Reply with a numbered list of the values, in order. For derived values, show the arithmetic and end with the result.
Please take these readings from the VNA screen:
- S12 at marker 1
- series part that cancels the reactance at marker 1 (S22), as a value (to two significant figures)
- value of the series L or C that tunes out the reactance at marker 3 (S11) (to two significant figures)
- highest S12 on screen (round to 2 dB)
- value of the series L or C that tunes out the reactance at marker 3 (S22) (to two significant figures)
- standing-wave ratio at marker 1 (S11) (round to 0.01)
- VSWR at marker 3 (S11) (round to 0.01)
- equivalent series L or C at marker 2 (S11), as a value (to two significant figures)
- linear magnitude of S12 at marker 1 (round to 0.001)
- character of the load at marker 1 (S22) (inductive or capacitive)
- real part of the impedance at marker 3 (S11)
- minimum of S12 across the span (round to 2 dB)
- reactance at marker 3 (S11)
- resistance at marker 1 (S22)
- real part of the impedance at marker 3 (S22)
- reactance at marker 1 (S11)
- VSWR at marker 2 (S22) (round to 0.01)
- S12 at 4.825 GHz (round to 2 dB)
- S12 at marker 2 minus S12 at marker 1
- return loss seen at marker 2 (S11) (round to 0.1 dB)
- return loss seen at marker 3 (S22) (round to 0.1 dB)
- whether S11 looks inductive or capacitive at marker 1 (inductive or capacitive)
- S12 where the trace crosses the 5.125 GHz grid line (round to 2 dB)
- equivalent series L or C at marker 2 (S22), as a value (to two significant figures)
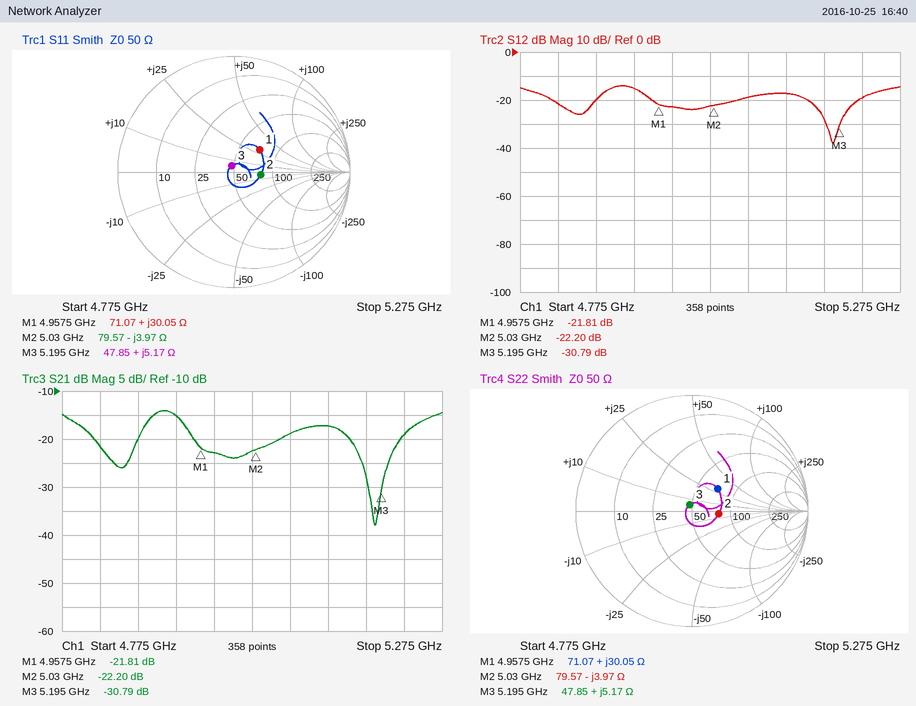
1. -21.81 dB
2. C = 1/(2π × 4.9575 GHz × 30.05 Ω) ≈ 1.1 pF
3. C = 1/(2π × 5.195 GHz × 5.17 Ω) ≈ 5.9 pF
4. -14 dB
5. C = 1/(2π × 5.195 GHz × 5.17 Ω) ≈ 5.9 pF
6. 1.83
7. 1.12
8. C = 1/(2π × 5.03 GHz × 3.97 Ω) ≈ 8.0 pF
9. 10^(-21.81/20) ≈ 0.081
10. inductive
11. 47.85 Ω
12. -38 dB
13. +5.17 Ω
14. 71.07 Ω
15. 47.85 Ω
16. +30.05 Ω
17. 1.60
18. -22 dB
19. -22.2 − (-21.81) = -0.39 dB
20. 12.8 dB
21. 24.9 dB
22. inductive
23. -18 dB
24. C = 1/(2π × 5.03 GHz × 3.97 Ω) ≈ 8.0 pF
